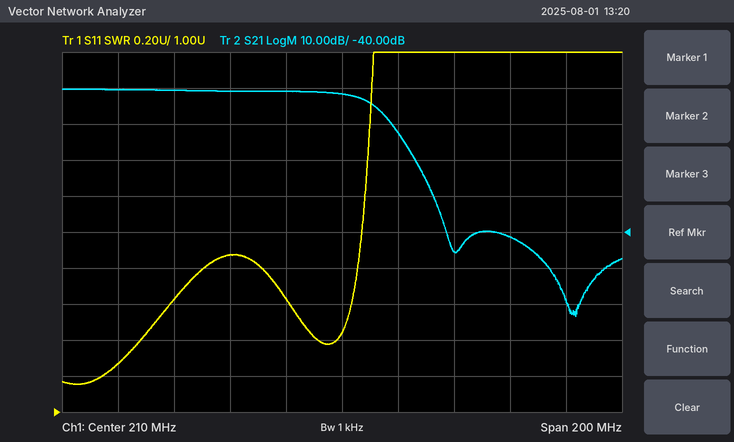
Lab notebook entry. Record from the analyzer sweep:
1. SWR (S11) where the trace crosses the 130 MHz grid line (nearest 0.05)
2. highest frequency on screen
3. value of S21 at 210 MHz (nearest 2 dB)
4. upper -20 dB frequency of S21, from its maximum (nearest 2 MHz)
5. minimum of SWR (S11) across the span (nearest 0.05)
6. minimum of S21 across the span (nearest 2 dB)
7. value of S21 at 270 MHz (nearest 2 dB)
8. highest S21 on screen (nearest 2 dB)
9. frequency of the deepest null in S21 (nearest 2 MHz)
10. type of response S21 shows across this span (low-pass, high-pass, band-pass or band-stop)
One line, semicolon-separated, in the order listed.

1.25; 310 MHz; -2 dB; 236 MHz; 1.15; -64 dB; -42 dB; 0 dB; 294 MHz; low-pass
